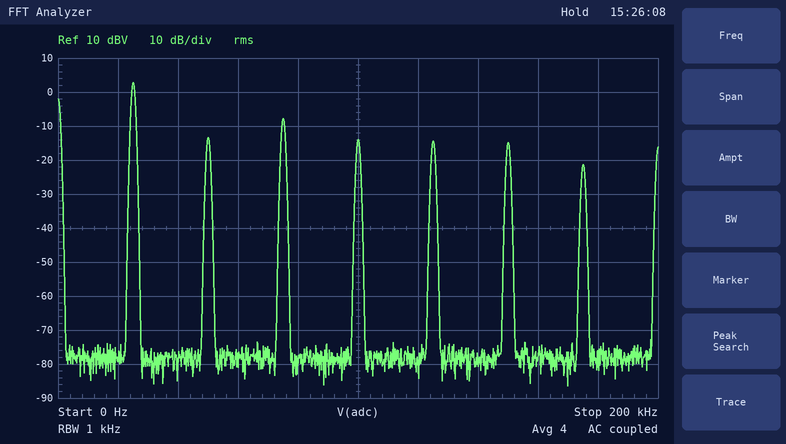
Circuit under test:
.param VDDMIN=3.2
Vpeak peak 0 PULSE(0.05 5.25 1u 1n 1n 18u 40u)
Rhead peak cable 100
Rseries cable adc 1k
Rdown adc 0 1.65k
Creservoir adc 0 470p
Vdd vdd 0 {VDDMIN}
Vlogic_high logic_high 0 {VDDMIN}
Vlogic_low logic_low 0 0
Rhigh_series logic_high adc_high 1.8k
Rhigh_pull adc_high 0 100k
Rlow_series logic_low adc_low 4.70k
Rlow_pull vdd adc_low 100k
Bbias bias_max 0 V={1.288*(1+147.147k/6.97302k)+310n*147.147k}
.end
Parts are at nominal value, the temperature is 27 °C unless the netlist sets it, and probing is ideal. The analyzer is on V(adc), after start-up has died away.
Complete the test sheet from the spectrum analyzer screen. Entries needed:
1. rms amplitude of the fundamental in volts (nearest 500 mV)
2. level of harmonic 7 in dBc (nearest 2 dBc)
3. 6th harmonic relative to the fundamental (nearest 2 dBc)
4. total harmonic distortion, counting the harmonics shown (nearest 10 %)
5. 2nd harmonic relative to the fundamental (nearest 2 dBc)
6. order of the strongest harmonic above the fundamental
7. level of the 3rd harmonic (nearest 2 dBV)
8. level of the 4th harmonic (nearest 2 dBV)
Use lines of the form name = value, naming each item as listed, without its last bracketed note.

rms amplitude of the fundamental in volts = 1.5 V
level of harmonic 7 in dBc = -24 dBc
6th harmonic relative to the fundamental = -18 dBc
total harmonic distortion, counting the harmonics shown = 40 %
2nd harmonic relative to the fundamental = -16 dBc
order of the strongest harmonic above the fundamental = 3
level of the 3rd harmonic = -8 dBV
level of the 4th harmonic = -14 dBV
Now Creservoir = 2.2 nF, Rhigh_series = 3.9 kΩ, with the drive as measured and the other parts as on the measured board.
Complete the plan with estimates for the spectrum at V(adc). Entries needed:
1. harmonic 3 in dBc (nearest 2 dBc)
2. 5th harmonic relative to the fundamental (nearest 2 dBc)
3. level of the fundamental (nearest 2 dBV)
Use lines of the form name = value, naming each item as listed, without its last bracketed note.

harmonic 3 in dBc = -12 dBc
5th harmonic relative to the fundamental = -20 dBc
level of the fundamental = 2 dBV
